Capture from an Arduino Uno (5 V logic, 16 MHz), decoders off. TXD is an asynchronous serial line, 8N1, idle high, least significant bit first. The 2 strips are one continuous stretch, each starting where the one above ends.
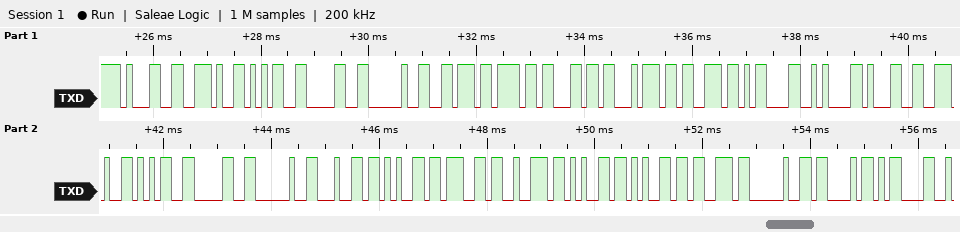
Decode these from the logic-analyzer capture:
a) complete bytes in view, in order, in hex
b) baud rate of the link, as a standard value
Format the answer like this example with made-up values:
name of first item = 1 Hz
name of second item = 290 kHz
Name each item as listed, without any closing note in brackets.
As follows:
complete bytes in view, in order, in hex = 31 2E 35 30 20 76 6F 6C 74 73 0D 0A 31 2E 35 30 20 64 65 67 72 65 65 73 20 43 0D
baud rate of the link, as a standard value = 9600 baud
